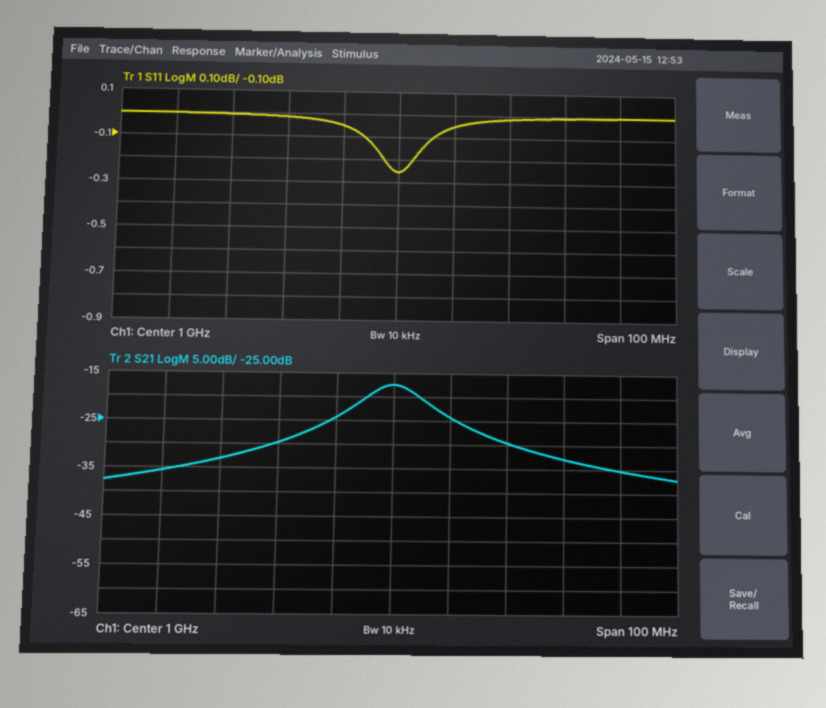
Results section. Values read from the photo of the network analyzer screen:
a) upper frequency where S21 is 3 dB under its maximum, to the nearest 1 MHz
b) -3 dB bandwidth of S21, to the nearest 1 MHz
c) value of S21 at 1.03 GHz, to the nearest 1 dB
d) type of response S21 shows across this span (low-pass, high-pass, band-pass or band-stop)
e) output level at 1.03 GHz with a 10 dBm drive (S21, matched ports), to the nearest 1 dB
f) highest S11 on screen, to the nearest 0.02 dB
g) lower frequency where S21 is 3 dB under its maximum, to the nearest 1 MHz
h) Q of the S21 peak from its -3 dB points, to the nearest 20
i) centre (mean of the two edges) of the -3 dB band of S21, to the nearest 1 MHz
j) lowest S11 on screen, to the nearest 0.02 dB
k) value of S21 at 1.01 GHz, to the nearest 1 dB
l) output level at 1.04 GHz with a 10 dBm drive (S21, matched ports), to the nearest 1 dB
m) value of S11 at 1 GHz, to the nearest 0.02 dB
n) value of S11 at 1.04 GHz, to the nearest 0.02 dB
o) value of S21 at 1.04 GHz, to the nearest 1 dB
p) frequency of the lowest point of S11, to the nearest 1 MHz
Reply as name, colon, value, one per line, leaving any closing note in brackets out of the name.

upper frequency where S21 is 3 dB under its maximum, to the nearest 1 MHz: 1.005 GHz
-3 dB bandwidth of S21, to the nearest 1 MHz: 10 MHz
value of S21 at 1.03 GHz, to the nearest 1 dB: -33 dB
type of response S21 shows across this span: band-pass
output level at 1.03 GHz with a 10 dBm drive (S21, matched ports), to the nearest 1 dB: -23 dBm
highest S11 on screen, to the nearest 0.02 dB: 0.00 dB
lower frequency where S21 is 3 dB under its maximum, to the nearest 1 MHz: 995 MHz
Q of the S21 peak from its -3 dB points, to the nearest 20: 100
centre (mean of the two edges) of the -3 dB band of S21, to the nearest 1 MHz: 1.000 GHz
lowest S11 on screen, to the nearest 0.02 dB: -0.26 dB
value of S21 at 1.01 GHz, to the nearest 1 dB: -24 dB
output level at 1.04 GHz with a 10 dBm drive (S21, matched ports), to the nearest 1 dB: -25 dBm
value of S11 at 1 GHz, to the nearest 0.02 dB: -0.26 dB
value of S11 at 1.04 GHz, to the nearest 0.02 dB: 0.00 dB
value of S21 at 1.04 GHz, to the nearest 1 dB: -35 dB
frequency of the lowest point of S11, to the nearest 1 MHz: 1.000 GHz
